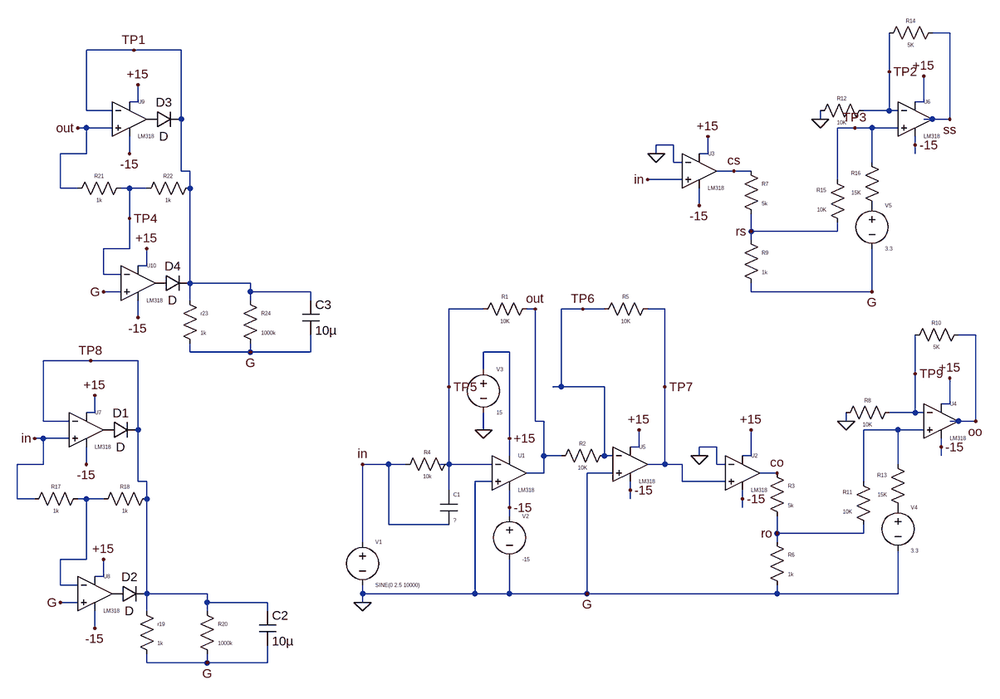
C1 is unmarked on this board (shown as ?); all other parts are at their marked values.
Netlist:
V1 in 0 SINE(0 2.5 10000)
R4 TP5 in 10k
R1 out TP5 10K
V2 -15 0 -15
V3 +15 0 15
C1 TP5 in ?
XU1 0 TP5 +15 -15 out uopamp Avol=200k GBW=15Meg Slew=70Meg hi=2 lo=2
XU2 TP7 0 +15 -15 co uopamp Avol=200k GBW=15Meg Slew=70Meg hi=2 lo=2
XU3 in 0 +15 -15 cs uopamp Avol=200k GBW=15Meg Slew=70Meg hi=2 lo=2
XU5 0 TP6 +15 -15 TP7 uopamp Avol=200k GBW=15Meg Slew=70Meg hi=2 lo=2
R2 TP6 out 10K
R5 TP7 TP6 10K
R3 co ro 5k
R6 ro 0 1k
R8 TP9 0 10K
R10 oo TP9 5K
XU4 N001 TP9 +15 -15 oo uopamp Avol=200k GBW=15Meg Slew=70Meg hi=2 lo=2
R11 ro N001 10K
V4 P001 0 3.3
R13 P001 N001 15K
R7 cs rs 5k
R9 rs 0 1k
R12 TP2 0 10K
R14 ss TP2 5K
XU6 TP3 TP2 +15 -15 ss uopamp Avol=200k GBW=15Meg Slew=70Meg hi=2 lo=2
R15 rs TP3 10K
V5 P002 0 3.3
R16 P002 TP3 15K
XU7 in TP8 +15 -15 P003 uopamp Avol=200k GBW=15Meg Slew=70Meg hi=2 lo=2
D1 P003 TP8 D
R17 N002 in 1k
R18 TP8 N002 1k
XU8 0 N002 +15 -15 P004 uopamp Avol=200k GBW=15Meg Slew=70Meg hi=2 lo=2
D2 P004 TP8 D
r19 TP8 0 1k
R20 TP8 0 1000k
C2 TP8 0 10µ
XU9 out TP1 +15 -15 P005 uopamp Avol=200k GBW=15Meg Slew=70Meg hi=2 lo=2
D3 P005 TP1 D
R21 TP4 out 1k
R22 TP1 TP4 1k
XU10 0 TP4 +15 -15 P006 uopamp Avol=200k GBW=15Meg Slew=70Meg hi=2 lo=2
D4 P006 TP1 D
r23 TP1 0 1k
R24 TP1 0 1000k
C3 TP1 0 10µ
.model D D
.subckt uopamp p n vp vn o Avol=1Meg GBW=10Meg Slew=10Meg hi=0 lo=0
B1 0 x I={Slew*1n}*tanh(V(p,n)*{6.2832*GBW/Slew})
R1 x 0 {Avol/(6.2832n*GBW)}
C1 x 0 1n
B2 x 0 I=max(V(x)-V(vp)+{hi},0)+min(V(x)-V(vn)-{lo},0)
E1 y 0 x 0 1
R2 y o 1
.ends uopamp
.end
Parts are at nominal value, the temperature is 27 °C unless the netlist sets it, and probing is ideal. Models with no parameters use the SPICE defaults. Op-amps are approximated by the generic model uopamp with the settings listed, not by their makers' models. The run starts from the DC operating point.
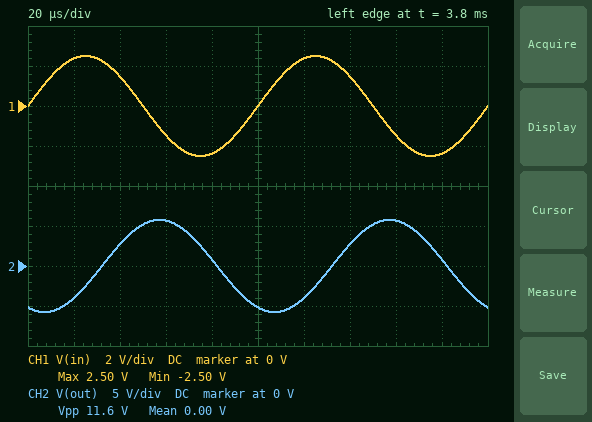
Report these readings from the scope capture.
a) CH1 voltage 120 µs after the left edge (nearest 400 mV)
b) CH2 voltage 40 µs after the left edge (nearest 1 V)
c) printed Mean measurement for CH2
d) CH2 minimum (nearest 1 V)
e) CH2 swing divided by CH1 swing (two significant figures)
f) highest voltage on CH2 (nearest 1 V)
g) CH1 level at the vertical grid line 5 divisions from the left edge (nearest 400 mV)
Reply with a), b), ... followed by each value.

a) 2.4 V
b) 3 V
c) 0.00 V
d) -6 V
e) 2.3
f) 6 V
g) 0 V
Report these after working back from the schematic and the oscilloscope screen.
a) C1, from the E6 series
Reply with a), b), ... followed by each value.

a) 3.3 nF
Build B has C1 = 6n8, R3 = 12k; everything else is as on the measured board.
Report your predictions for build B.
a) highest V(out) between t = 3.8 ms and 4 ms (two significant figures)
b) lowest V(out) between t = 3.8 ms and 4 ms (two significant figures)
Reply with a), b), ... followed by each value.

a) 11 V
b) -11 V
